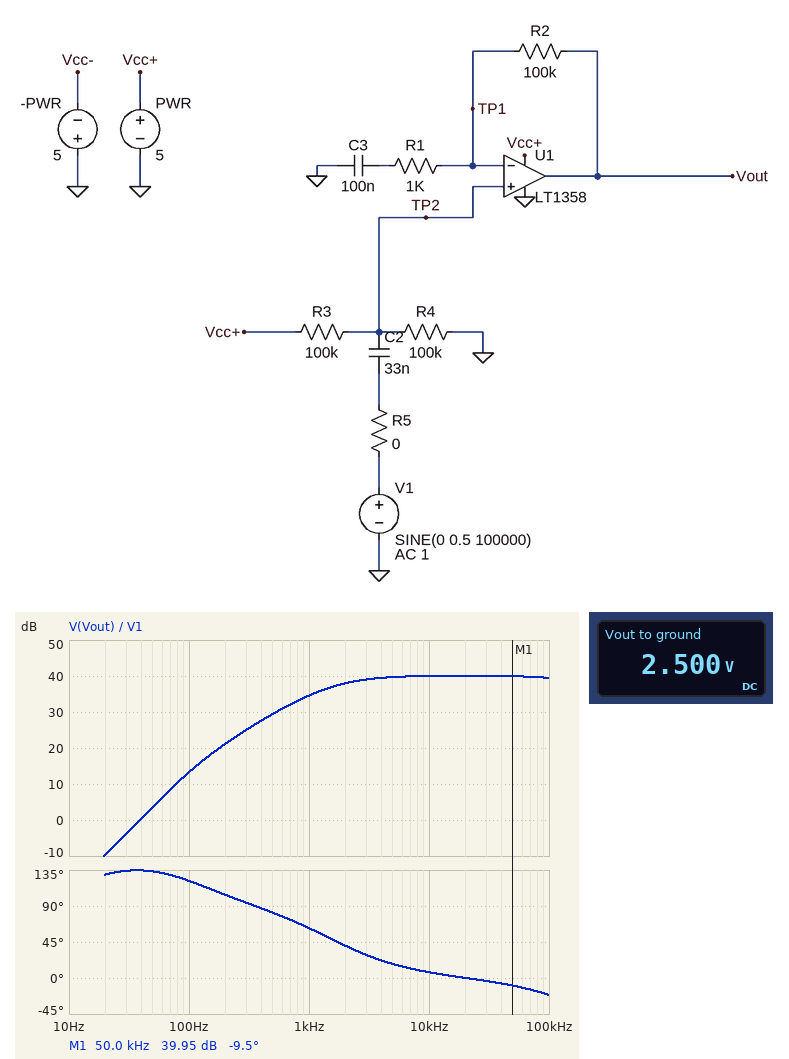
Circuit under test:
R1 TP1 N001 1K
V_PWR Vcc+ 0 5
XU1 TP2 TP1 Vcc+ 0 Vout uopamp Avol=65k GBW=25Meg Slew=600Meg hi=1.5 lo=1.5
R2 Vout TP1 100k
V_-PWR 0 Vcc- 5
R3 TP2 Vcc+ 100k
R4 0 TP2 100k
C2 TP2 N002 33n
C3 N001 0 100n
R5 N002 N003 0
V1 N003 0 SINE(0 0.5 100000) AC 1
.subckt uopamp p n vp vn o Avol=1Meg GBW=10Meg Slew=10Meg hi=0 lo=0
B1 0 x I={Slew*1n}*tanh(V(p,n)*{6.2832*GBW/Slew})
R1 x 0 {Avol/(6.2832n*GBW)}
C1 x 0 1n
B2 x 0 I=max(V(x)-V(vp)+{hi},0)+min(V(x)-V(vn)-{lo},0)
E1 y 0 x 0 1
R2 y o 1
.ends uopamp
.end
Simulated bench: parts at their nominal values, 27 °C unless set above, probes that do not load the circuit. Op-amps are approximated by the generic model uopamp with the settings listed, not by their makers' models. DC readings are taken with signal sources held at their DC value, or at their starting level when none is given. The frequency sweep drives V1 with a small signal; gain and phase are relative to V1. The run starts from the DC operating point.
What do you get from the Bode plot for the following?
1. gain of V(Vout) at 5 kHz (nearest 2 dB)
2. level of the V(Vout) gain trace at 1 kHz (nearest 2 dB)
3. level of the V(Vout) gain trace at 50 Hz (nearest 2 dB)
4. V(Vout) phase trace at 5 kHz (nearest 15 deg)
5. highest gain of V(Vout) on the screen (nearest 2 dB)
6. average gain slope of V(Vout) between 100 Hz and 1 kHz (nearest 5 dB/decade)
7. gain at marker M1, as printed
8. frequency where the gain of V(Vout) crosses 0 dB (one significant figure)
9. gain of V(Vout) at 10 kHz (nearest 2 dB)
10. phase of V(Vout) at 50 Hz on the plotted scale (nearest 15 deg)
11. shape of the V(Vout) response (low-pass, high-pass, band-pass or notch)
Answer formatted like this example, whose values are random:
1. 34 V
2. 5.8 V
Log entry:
1. 40 dB
2. 34 dB
3. 4 dB
4. 15 deg
5. 40 dB
6. 20 dB/decade
7. 39.95 dB
8. 40 Hz
9. 40 dB
10. 135 deg
11. high-pass
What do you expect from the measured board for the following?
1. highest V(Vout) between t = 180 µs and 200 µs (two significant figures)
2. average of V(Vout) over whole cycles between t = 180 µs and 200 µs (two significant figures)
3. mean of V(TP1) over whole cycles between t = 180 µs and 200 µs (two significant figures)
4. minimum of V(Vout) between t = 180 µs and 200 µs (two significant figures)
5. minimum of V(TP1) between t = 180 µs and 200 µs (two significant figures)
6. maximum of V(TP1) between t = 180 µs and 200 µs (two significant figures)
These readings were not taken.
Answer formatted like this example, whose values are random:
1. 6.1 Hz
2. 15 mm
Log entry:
1. 3.6 V
2. 2.5 V
3. 2.5 V
4. 1.4 V
5. 2.5 V
6. 2.5 V
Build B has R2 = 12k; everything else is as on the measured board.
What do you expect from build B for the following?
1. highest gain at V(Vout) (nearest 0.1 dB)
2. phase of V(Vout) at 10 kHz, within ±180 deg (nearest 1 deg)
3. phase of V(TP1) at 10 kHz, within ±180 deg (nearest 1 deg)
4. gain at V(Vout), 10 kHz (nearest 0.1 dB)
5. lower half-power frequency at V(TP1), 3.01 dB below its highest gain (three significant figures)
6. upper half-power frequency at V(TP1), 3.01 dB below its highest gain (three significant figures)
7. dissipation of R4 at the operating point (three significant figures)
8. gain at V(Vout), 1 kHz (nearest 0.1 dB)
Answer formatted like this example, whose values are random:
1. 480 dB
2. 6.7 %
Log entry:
1. 22.3 dB
2. 9 deg
3. 0 deg
4. 22.2 dB
5. 96.6 Hz
6. 1.92 MHz
7. 62.5 µW
8. 16.8 dB
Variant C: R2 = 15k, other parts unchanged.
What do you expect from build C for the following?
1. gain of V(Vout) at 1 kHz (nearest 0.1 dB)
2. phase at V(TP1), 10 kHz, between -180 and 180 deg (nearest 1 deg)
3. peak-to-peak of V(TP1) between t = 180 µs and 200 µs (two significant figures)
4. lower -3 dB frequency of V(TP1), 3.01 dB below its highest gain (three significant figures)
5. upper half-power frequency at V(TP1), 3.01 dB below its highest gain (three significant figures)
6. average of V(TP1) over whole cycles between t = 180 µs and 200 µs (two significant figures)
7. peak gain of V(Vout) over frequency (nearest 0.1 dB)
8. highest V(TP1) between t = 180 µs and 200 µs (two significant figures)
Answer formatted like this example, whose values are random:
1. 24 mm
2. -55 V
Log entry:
1. 18.6 dB
2. 0 deg
3. 130 mV
4. 96.6 Hz
5. 1.56 MHz
6. 2.5 V
7. 24.1 dB
8. 2.6 V
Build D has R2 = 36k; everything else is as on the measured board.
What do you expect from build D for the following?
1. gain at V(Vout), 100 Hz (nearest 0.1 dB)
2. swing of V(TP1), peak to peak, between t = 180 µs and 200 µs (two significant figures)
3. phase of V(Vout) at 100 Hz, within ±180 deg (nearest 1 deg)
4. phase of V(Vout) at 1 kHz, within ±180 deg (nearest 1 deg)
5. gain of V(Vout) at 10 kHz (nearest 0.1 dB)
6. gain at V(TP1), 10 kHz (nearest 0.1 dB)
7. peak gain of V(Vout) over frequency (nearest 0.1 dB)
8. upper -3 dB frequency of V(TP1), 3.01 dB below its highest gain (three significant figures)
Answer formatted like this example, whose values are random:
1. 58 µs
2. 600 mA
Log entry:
1. 5.2 dB
2. 58 mV
3. 107 deg
4. 61 deg
5. 31.3 dB
6. 0 dB
7. 31.4 dB
8. 675 kHz
